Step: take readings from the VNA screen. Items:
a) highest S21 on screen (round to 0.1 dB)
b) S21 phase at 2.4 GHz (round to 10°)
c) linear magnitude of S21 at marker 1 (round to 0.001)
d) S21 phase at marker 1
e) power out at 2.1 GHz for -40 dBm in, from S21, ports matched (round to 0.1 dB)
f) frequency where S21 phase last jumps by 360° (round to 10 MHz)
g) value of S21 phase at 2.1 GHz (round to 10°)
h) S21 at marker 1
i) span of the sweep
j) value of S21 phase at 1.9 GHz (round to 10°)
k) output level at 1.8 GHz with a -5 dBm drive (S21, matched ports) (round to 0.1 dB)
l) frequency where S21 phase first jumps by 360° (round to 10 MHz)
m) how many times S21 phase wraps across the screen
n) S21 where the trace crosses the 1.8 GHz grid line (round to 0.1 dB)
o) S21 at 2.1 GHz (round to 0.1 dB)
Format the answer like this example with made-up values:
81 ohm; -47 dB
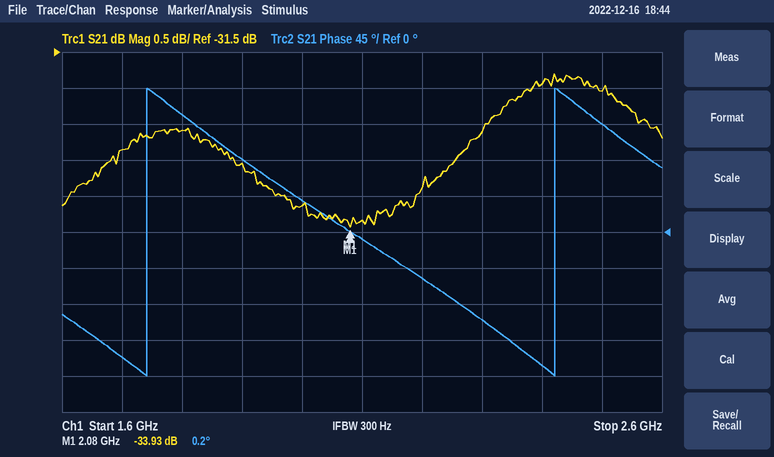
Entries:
-31.8 dB; -170°; 0.020; 0.2°; -73.8 dBm; 2.42 GHz; -10°; -33.93 dB; 1 GHz; 90°; -37.6 dBm; 1.74 GHz; 2; -32.6 dB; -33.8 dB
